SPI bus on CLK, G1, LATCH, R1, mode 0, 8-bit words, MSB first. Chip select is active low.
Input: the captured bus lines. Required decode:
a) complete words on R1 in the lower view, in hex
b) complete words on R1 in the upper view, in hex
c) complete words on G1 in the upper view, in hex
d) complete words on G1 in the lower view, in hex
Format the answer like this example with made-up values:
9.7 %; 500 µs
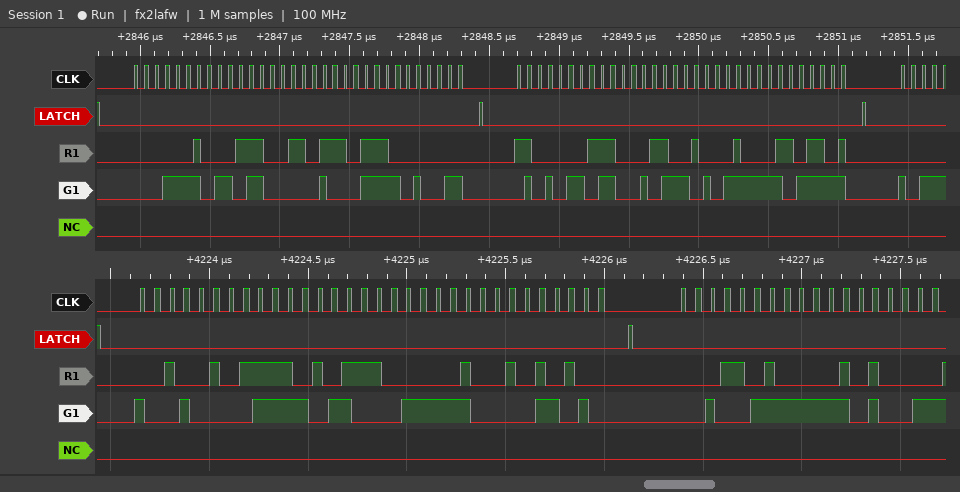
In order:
25, EB, 82, 54, 1A, 14; 02, 39, BB, 80, C1, C6, 44, 6D; 1E, D8, 23, D3, 56, CB, AF, DF; 90, F6, 3E, 1A, 27, F4
